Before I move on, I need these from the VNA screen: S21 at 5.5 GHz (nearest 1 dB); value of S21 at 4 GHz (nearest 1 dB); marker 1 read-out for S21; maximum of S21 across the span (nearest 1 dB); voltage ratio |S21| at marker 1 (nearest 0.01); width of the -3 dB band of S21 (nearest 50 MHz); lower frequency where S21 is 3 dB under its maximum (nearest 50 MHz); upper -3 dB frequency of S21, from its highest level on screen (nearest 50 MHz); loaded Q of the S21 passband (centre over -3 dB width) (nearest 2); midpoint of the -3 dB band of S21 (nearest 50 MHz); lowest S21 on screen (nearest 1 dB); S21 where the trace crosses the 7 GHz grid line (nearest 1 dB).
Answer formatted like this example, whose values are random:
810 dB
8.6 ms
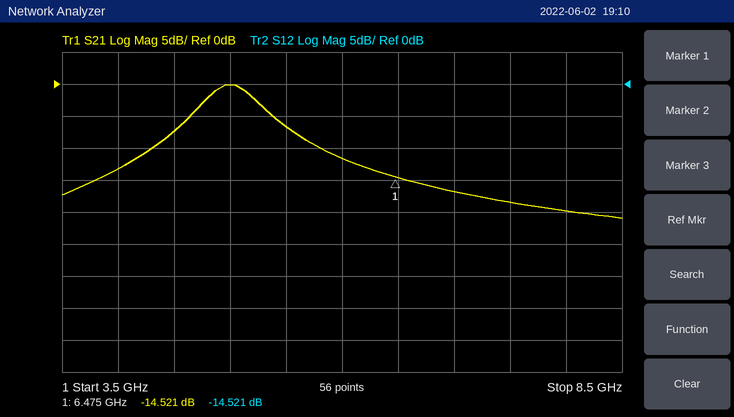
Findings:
-7 dB
-13 dB
-14.521 dB
0 dB
0.19
500 MHz
4.75 GHz
5.25 GHz
10
5.00 GHz
-21 dB
-17 dB
